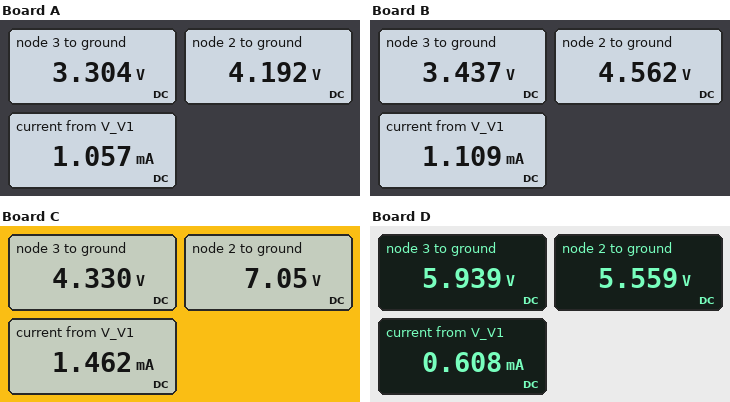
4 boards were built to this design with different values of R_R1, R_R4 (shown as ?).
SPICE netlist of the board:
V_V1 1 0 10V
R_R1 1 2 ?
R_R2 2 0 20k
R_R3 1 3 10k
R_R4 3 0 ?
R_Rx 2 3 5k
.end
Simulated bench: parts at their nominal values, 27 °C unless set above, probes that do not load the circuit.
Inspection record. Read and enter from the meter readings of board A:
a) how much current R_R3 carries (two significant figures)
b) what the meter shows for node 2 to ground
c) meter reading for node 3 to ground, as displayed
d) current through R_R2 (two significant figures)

670 µA
4.192 V
3.304 V
210 µA
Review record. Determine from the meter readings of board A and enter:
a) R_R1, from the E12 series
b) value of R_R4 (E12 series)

15 kΩ
3.9 kΩ
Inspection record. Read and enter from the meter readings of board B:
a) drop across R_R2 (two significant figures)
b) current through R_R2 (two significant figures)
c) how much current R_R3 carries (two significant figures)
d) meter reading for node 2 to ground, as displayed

4.6 V
230 µA
660 µA
4.562 V
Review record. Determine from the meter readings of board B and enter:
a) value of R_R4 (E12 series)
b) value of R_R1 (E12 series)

3.9 kΩ
12 kΩ
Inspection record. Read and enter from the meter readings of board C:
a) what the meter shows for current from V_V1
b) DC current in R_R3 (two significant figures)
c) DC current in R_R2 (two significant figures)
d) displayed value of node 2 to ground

1.462 mA
570 µA
350 µA
7.05 V
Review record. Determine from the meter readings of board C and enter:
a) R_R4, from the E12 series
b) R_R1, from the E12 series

3.9 kΩ
3.3 kΩ
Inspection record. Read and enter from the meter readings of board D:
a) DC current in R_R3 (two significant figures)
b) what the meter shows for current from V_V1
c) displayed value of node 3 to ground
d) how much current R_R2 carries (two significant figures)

410 µA
0.608 mA
5.939 V
280 µA
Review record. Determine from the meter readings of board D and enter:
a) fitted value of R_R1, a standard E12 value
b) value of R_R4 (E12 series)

22 kΩ
18 kΩ
